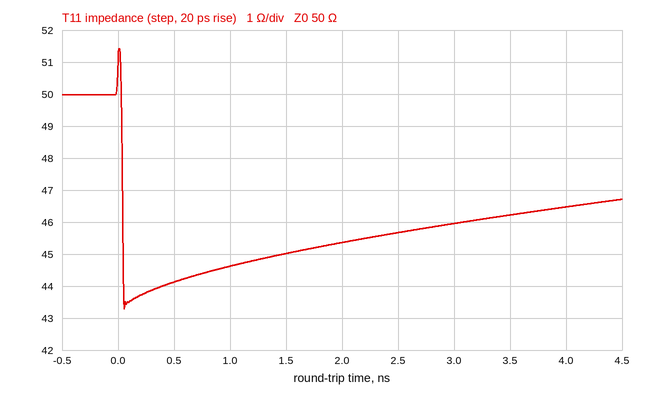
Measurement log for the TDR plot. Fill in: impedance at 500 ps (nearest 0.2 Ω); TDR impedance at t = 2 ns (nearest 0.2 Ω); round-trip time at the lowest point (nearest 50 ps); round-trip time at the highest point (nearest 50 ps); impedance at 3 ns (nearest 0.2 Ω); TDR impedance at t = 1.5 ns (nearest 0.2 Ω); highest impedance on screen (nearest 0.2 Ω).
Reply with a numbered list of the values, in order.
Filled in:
1. 44.2 Ω
2. 45.4 Ω
3. 50 ps
4. 0 ps
5. 46.0 Ω
6. 45.0 Ω
7. 51.4 Ω
